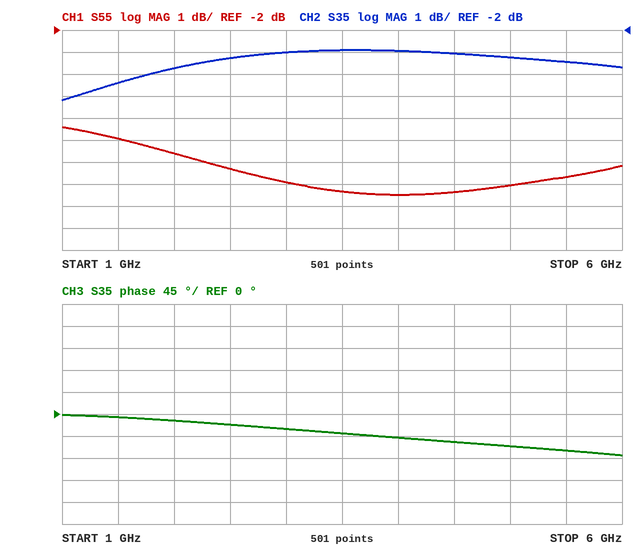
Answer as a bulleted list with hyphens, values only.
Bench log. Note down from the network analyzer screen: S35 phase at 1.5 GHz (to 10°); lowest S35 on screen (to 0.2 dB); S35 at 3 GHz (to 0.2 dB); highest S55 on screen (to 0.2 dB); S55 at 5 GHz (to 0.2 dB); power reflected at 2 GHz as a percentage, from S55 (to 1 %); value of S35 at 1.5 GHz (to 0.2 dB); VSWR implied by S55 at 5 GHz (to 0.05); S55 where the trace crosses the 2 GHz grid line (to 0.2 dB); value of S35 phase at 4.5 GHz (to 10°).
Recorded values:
- -10°
- -5.2 dB
- -3.0 dB
- -6.4 dB
- -9.0 dB
- 17 %
- -4.4 dB
- 2.10
- -7.6 dB
- -60°
